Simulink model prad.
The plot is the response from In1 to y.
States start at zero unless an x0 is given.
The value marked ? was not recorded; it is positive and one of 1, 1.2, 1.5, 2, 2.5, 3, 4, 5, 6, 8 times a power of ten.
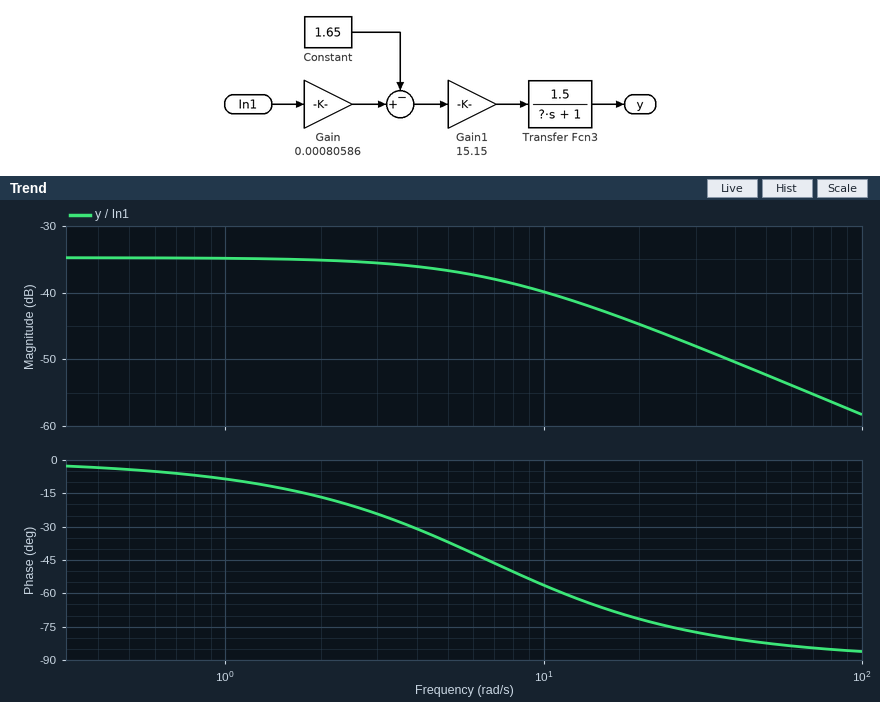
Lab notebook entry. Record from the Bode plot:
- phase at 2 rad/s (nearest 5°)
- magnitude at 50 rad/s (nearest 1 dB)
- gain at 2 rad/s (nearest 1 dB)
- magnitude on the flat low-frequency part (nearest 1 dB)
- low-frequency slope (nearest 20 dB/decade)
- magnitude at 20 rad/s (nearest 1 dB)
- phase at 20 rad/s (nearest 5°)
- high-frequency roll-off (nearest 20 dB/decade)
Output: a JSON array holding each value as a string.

["-15°", "-52 dB", "-35 dB", "-35 dB", "0 dB/decade", "-45 dB", "-70°", "-20 dB/decade"]
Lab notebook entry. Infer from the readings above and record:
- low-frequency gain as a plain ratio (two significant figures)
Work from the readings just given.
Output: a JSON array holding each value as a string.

["0.018"]
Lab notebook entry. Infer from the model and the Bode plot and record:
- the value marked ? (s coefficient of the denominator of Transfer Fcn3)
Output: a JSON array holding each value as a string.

["0.15"]
